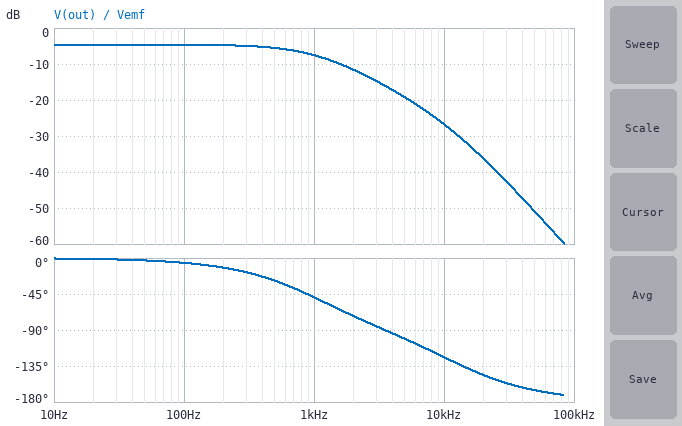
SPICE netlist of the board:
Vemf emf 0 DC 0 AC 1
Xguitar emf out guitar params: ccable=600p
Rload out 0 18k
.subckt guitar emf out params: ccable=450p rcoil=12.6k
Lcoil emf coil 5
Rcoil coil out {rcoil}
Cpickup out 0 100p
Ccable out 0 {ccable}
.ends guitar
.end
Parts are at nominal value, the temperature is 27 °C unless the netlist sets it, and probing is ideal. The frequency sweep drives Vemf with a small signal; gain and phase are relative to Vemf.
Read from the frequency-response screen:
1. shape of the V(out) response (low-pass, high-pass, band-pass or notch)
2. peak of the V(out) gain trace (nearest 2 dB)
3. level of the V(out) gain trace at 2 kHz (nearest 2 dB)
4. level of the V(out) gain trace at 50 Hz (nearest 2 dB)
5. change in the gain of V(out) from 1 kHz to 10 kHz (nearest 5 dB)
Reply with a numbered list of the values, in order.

1. low-pass
2. -4 dB
3. -12 dB
4. -4 dB
5. -20 dB
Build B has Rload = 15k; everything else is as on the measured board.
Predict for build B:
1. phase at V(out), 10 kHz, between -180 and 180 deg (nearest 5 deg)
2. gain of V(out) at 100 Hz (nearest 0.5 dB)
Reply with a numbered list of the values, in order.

1. -120 deg
2. -5.5 dB
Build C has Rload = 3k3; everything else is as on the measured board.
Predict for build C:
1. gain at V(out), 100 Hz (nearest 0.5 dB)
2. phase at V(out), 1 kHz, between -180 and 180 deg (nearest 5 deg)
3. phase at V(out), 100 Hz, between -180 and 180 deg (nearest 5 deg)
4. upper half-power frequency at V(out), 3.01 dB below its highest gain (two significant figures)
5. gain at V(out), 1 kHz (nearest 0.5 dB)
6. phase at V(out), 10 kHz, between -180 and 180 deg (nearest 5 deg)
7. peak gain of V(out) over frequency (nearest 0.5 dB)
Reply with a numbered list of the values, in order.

1. -14.0 dB
2. -65 deg
3. -10 deg
4. 510 Hz
5. -20.5 dB
6. -95 deg
7. -13.5 dB
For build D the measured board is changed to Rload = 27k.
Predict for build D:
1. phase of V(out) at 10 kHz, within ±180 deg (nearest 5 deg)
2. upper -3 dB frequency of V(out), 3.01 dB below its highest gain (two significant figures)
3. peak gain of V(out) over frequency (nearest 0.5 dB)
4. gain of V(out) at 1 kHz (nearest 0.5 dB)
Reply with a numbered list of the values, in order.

1. -135 deg
2. 1.4 kHz
3. -3.5 dB
4. -5.0 dB
